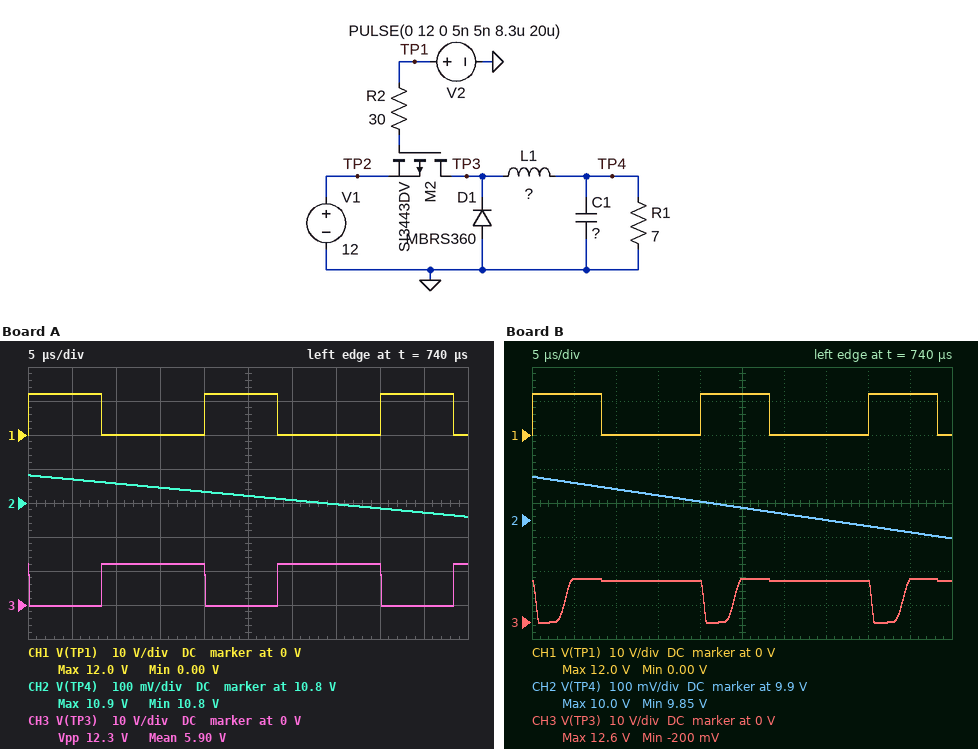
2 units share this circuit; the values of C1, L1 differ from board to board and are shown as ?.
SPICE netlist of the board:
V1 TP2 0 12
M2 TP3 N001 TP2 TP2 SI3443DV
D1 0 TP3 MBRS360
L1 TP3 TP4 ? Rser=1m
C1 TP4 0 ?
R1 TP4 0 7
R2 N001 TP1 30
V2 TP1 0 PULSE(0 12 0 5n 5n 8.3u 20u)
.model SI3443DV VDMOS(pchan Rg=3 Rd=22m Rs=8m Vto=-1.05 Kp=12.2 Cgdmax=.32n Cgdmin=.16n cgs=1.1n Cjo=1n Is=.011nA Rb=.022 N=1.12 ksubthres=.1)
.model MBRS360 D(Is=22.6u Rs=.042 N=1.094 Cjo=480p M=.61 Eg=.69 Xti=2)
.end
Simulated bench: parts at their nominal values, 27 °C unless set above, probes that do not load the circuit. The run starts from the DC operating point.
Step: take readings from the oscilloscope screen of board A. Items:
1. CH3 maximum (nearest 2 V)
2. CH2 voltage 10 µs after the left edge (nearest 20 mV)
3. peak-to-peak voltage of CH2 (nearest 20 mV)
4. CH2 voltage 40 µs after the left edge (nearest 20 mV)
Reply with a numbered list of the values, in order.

1. 12 V
2. 10.86 V
3. 120 mV
4. 10.78 V
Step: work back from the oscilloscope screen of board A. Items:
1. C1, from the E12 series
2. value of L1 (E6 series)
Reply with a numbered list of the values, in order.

1. 150 µF
2. 6.8 mH
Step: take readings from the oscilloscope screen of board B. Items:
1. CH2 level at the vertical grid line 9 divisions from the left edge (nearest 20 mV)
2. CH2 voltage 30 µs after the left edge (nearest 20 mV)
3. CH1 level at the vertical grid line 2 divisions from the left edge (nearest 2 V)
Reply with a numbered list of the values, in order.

1. 9.86 V
2. 9.92 V
3. 0 V
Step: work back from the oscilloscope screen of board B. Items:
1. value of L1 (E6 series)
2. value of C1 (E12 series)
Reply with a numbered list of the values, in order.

1. 1.5 mH
2. 390 µF
